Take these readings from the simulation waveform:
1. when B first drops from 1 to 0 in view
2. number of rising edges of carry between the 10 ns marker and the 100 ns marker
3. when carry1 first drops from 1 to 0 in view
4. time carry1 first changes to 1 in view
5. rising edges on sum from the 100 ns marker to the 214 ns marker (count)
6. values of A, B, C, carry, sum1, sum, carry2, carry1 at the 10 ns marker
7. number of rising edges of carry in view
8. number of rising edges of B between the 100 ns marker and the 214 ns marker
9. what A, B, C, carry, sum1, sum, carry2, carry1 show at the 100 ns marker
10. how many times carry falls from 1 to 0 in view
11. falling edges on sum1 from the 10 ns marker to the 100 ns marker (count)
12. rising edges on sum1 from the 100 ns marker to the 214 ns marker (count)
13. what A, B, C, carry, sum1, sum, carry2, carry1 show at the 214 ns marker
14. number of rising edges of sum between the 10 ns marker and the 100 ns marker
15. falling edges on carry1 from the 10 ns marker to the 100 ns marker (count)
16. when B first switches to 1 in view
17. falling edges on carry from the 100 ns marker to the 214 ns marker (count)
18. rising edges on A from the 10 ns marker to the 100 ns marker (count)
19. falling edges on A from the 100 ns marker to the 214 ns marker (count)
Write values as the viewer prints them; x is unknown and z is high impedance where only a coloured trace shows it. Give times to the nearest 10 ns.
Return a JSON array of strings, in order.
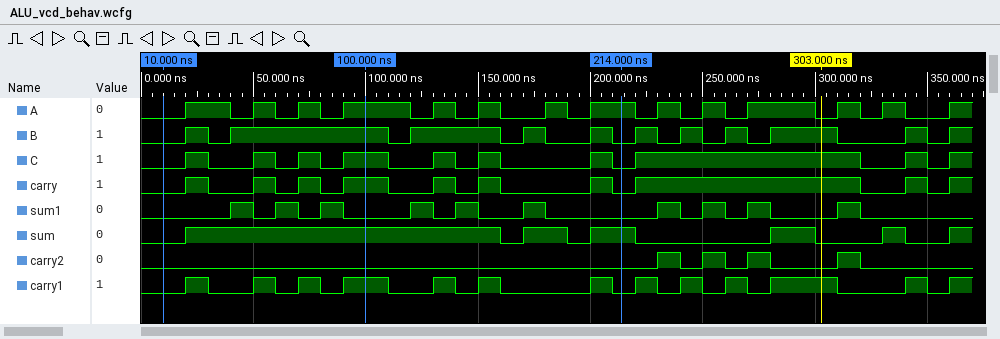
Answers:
["30 ns", "4", "30 ns", "20 ns", "2", "A=0, B=0, C=0, carry=0, sum1=0, sum=0, carry2=0, carry1=0", "10", "3", "A=1, B=1, C=1, carry=1, sum1=0, sum=1, carry2=0, carry1=1", "9", "3", "3", "A=1, B=0, C=0, carry=0, sum1=0, sum=1, carry2=0, carry1=0", "1", "3", "20 ns", "4", "4", "4"]
